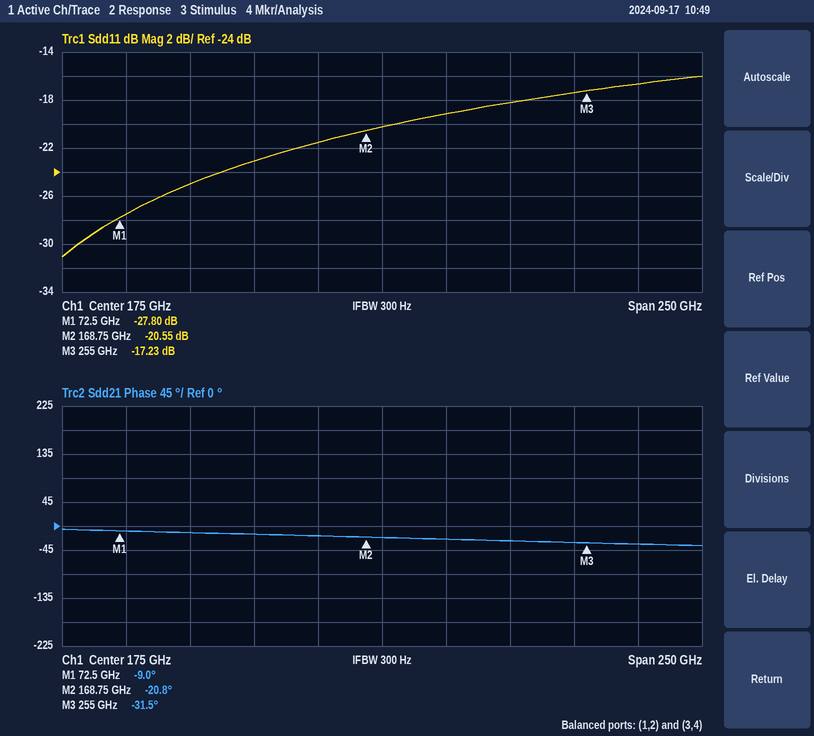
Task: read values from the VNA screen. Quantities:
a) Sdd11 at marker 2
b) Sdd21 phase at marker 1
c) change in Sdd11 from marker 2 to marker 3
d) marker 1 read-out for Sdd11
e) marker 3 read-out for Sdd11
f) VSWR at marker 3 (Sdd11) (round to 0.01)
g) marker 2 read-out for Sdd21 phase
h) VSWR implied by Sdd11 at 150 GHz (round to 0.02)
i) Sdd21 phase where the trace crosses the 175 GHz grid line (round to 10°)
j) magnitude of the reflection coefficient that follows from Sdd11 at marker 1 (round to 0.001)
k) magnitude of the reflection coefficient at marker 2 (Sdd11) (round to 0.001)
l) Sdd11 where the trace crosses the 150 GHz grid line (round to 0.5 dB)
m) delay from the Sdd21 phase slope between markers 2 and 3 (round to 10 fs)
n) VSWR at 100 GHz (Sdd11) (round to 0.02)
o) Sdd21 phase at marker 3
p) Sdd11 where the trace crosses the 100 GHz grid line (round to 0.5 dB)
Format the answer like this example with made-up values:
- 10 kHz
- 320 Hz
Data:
- -20.55 dB
- -9.0°
- 3.32 dB
- -27.80 dB
- -17.23 dB
- 1.32
- -20.8°
- 1.18
- -20°
- 0.041
- 0.094
- -21.5 dB
- 340 fs
- 1.12
- -31.5°
- -25.0 dB
